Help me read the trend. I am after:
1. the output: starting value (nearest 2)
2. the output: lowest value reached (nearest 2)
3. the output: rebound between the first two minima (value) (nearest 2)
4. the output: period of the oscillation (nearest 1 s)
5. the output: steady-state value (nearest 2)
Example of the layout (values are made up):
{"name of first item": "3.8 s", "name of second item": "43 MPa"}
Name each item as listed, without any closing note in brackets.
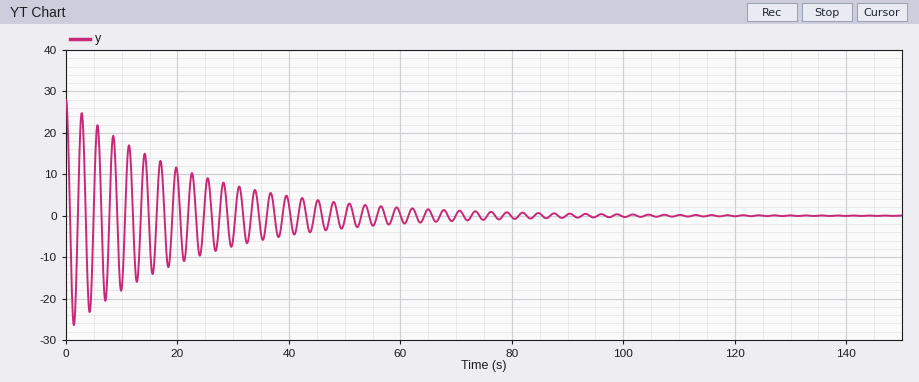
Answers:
{"the output: starting value": "28", "the output: lowest value reached": "-26", "the output: rebound between the first two minima (value)": "24", "the output: period of the oscillation": "3 s", "the output: steady-state value": "0"}
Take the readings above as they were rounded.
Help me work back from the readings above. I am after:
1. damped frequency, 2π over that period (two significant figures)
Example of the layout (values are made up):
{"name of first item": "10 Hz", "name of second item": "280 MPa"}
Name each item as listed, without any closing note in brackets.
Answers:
{"damped frequency, 2π over that period": "2.1 rad/s"}
